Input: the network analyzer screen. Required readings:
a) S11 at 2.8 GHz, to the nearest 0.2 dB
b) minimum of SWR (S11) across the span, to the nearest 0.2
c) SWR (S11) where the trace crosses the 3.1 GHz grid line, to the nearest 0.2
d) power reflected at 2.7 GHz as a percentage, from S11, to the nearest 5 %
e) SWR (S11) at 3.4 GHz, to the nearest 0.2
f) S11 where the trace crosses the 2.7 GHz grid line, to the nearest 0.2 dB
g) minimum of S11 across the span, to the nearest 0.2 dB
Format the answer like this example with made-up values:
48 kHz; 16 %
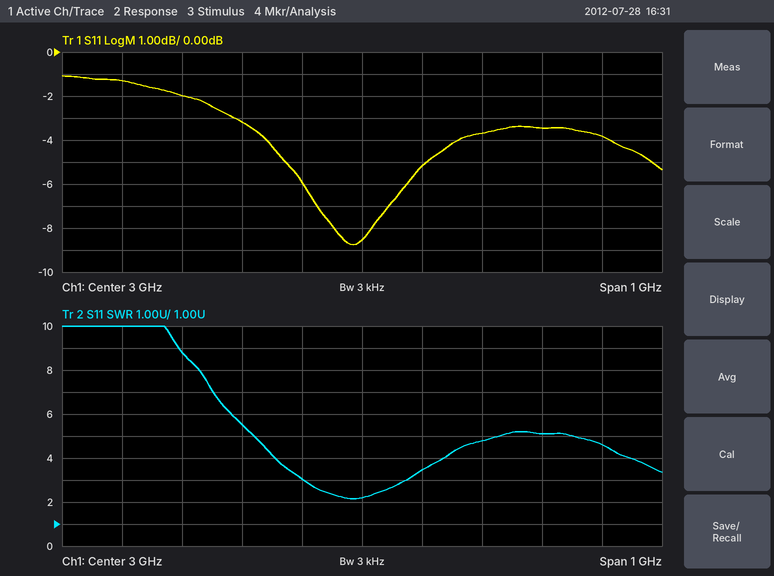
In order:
-3.2 dB; 2.2; 3.4; 65 %; 4.6; -2.0 dB; -8.8 dB
